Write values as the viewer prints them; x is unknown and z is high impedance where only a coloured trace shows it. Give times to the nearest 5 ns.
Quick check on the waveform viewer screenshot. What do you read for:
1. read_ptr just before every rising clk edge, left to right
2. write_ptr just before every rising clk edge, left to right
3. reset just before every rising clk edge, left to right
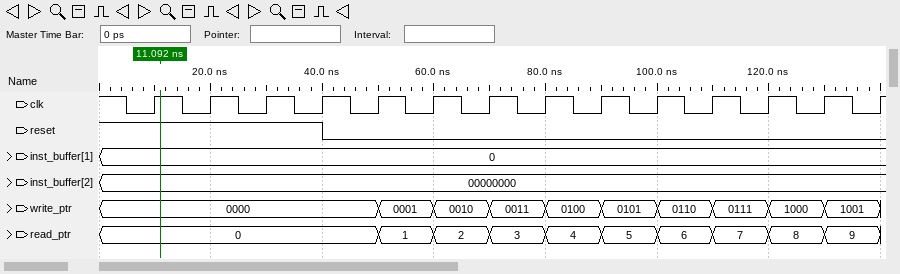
0, 0, 0, 0, 0, 1, 2, 3, 4, 5, 6, 7, 8, 9
0000, 0000, 0000, 0000, 0000, 0001, 0010, 0011, 0100, 0101, 0110, 0111, 1000, 1001
1 1 1 1 0 0 0 0 0 0 0 0 0 0
